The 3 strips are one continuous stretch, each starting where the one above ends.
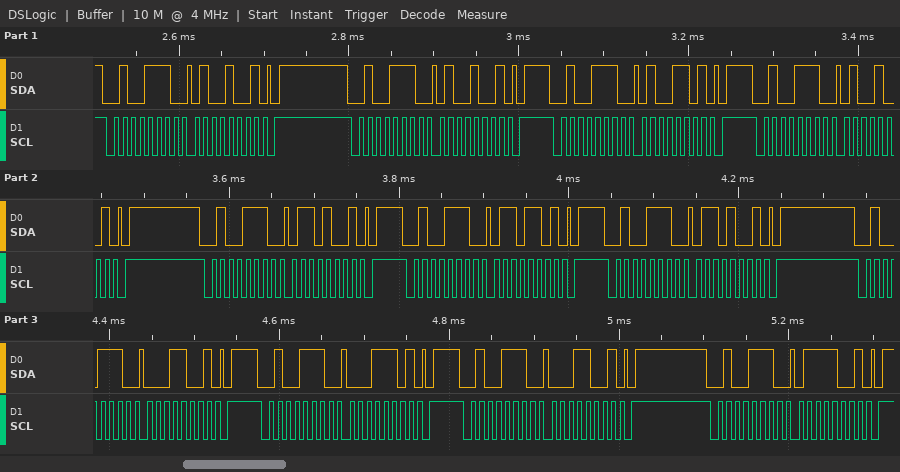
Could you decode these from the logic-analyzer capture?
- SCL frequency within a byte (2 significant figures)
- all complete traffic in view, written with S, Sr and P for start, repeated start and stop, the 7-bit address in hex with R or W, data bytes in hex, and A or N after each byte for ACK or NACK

100 kHz
S 27W A 49 A P S 27W A 49 A P S 27W A 4D A P S 27W A 49 A P S 27W A 69 A P S 27W A 6D A P S 27W A 69 A P S 27W A 19 A P S 27W A 1D A P S 27W A 19 A P S 27W A 79 A P
